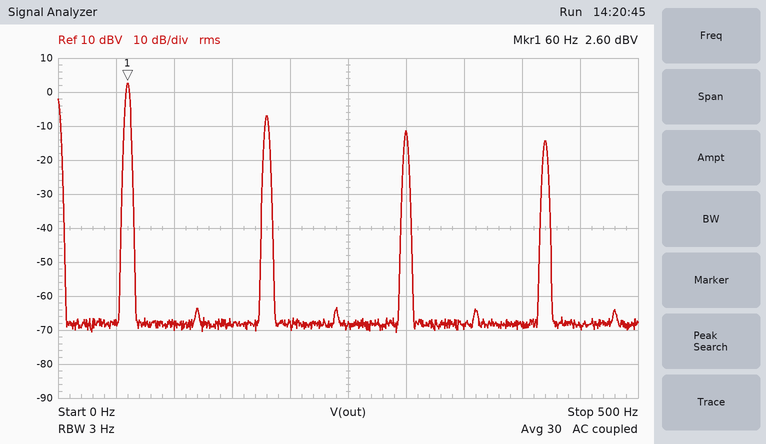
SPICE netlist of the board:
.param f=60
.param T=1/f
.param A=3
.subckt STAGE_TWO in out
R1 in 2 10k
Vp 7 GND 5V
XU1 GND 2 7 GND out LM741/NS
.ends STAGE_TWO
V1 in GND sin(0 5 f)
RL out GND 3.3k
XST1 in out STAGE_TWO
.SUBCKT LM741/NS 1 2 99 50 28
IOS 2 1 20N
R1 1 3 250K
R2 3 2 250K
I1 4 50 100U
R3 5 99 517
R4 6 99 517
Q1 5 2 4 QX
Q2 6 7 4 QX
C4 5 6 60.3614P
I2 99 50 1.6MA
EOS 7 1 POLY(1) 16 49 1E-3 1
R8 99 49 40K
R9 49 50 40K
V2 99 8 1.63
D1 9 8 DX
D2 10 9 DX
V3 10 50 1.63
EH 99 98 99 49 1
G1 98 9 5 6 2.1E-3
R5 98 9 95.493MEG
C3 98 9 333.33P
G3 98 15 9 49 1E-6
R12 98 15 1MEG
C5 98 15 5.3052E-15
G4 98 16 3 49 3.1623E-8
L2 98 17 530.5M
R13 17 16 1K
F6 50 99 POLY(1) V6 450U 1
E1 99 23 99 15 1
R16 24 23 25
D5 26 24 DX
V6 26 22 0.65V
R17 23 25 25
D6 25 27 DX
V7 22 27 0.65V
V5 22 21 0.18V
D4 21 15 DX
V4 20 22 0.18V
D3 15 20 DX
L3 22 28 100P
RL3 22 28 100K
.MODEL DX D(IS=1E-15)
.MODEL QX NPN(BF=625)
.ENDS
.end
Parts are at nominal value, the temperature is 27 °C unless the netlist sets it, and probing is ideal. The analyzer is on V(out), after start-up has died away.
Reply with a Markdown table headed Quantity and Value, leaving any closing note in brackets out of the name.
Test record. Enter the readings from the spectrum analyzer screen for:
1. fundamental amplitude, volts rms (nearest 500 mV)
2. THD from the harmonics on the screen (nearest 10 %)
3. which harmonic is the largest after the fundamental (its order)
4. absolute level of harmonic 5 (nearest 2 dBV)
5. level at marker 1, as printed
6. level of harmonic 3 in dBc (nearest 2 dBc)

| Quantity | Value |
|---|---|
| fundamental amplitude, volts rms | 1.5 V |
| THD from the harmonics on the screen | 40 % |
| which harmonic is the largest after the fundamental | 3 |
| absolute level of harmonic 5 | -12 dBV |
| level at marker 1, as printed | 2.60 dBV |
| level of harmonic 3 in dBc | -10 dBc |
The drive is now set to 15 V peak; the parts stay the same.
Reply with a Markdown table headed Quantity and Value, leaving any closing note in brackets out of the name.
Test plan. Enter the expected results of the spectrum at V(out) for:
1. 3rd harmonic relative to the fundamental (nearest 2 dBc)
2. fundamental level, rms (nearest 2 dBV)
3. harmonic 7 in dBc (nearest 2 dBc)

| Quantity | Value |
|---|---|
| 3rd harmonic relative to the fundamental | 10 dBc |
| fundamental level, rms | -18 dBV |
| harmonic 7 in dBc | 10 dBc |
